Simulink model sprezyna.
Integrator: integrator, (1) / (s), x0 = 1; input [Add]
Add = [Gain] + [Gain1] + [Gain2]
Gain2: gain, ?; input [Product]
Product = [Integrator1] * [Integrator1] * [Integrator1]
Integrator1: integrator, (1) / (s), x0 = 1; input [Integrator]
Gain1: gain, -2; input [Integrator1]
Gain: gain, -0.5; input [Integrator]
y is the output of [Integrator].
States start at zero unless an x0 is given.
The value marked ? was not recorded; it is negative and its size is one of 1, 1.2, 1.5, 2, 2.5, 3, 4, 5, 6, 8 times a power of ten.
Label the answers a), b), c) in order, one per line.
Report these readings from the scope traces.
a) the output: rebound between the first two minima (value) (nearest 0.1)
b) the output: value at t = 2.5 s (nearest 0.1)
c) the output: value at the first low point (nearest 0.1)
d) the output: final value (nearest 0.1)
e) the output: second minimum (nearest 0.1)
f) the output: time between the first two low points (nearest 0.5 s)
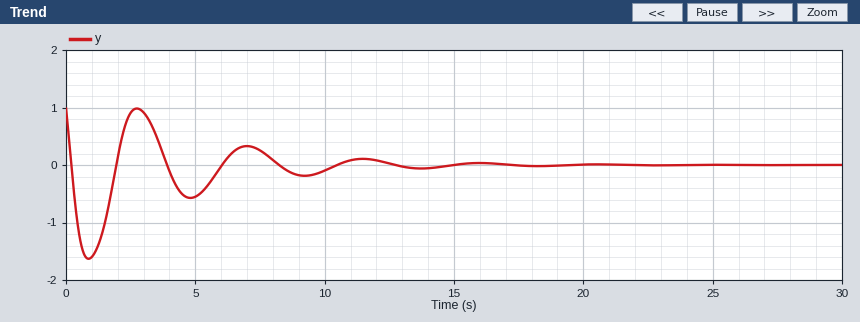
a) 1.0
b) 0.9
c) -1.6
d) 0.0
e) -0.6
f) 4.0 s
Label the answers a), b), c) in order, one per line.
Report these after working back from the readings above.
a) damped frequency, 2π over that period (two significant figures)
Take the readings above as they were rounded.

a) 1.6 rad/s
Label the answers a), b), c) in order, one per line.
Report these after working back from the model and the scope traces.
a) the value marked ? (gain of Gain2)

a) -2
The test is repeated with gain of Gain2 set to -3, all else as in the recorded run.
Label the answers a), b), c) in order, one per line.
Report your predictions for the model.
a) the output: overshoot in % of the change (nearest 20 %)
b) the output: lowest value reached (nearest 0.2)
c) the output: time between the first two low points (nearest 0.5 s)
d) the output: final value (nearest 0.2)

a) 180 %
b) -1.8
c) 3.5 s
d) 0.0
